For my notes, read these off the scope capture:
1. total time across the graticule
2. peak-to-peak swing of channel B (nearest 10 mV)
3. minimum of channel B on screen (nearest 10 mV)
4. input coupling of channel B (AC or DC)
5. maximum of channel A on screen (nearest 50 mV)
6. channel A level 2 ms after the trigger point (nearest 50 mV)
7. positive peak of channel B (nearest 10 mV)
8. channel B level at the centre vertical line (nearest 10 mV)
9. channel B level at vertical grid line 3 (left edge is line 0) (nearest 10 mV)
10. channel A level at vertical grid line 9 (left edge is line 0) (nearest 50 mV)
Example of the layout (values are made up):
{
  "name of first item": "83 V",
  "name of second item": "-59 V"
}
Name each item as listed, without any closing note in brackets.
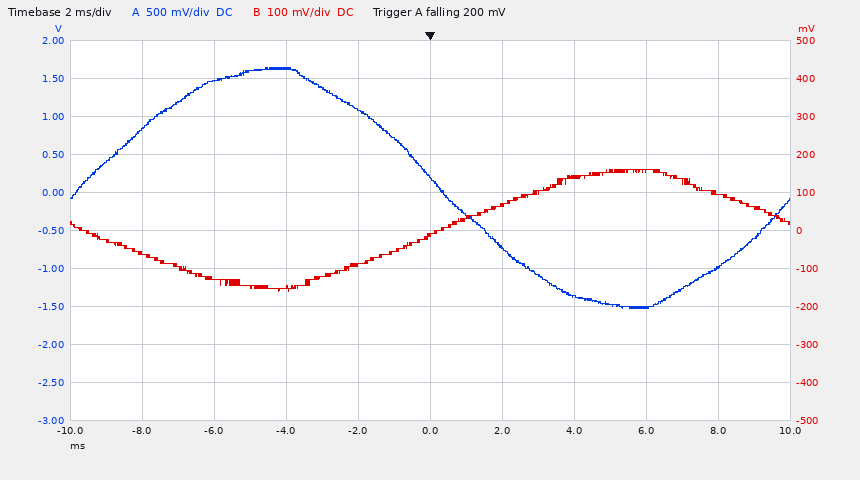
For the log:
{
  "total time across the graticule": "20 ms",
  "peak-to-peak swing of channel B": "320 mV",
  "minimum of channel B on screen": "-160 mV",
  "input coupling of channel B": "DC",
  "maximum of channel A on screen": "1.65 V",
  "channel A level 2 ms after the trigger point": "-700 mV",
  "positive peak of channel B": "160 mV",
  "channel B level at the centre vertical line": "-20 mV",
  "channel B level at vertical grid line 3 (left edge is line 0)": "-150 mV",
  "channel A level at vertical grid line 9 (left edge is line 0)": "-1.00 V"
}
